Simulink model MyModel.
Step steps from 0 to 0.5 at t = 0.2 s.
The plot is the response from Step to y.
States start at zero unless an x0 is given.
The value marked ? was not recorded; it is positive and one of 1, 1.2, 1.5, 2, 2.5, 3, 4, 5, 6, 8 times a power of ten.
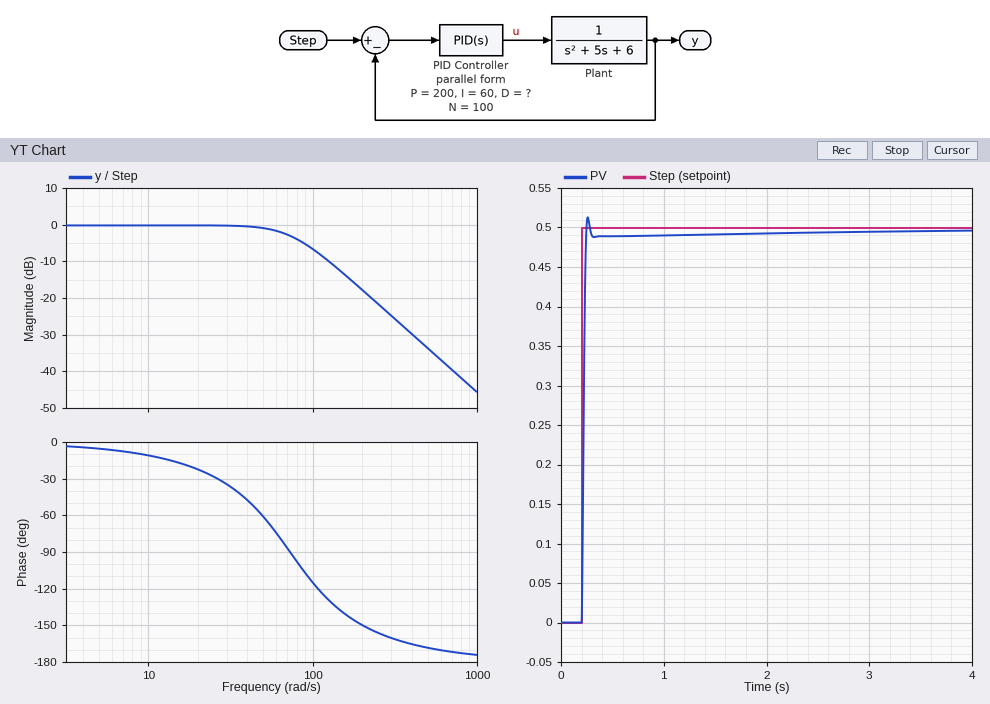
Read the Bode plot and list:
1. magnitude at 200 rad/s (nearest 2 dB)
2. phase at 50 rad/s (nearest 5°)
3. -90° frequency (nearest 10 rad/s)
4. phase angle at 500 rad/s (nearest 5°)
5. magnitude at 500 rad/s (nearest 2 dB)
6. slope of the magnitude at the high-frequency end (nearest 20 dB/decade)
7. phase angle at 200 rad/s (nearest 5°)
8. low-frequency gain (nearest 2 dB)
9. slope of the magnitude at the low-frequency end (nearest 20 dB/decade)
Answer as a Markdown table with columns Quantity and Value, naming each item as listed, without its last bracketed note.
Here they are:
| Quantity | Value |
|---|---|
| magnitude at 200 rad/s | -18 dB |
| phase at 50 rad/s | -60° |
| -90° frequency | 70 rad/s |
| phase angle at 500 rad/s | -170° |
| magnitude at 500 rad/s | -34 dB |
| slope of the magnitude at the high-frequency end | -40 dB/decade |
| phase angle at 200 rad/s | -150° |
| low-frequency gain | 0 dB |
| slope of the magnitude at the low-frequency end | 0 dB/decade |
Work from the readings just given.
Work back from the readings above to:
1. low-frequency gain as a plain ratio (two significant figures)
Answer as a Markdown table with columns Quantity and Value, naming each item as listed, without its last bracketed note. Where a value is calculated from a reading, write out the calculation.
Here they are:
| Quantity | Value |
|---|---|
| low-frequency gain as a plain ratio | 10^(0 / 20) = 1.0 |
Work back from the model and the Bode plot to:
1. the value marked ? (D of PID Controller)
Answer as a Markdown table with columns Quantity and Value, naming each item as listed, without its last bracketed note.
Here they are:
| Quantity | Value |
|---|---|
| the value marked ? | 50 |
